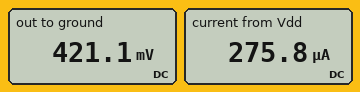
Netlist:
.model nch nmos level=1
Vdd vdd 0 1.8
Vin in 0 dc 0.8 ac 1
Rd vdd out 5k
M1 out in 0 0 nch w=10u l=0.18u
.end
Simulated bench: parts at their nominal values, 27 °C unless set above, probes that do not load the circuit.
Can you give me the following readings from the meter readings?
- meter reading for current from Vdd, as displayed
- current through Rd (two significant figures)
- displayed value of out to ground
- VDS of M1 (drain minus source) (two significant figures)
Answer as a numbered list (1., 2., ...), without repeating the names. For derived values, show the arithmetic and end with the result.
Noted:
1. 275.8 µA
2. (1.8 V - 421.1 mV) / 5 kΩ = 280 µA
3. 421.1 mV
4. 421.1 mV = 420 mV
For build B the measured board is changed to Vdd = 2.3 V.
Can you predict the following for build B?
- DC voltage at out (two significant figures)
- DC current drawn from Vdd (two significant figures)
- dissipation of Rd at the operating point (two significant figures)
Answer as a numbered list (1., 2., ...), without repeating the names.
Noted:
1. 620 mV
2. 340 µA
3. 570 µW
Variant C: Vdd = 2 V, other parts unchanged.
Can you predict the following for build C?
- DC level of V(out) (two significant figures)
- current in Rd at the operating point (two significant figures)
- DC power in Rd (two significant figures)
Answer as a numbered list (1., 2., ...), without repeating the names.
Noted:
1. 490 mV
2. 300 µA
3. 460 µW
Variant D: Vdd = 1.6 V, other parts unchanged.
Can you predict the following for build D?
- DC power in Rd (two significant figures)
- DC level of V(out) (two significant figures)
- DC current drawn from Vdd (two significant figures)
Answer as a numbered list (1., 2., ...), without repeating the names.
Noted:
1. 310 µW
2. 360 mV
3. 250 µA
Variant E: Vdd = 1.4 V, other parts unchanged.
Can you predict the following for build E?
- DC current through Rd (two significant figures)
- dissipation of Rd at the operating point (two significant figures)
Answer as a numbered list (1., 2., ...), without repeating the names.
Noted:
1. 220 µA
2. 240 µW
